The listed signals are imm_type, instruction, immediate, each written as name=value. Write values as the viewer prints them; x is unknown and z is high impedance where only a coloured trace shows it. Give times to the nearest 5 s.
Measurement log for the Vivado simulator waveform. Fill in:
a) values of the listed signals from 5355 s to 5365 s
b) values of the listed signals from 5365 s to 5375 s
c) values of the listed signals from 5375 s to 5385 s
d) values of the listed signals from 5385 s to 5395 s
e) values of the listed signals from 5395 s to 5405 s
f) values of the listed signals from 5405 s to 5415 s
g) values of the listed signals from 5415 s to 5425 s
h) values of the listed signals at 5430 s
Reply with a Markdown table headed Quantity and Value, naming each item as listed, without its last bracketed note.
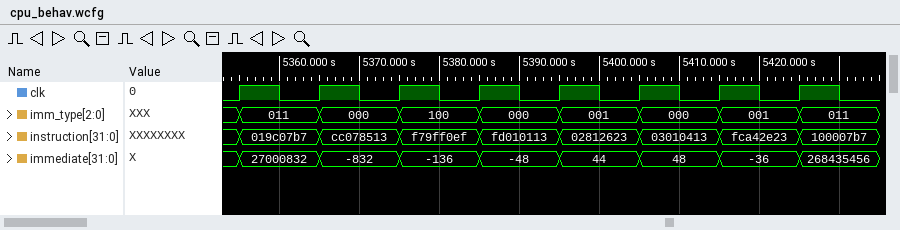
| Quantity | Value |
|---|---|
| values of the listed signals from 5355 s to 5365 s | imm_type=011, instruction=019c07b7, immediate=27000832 |
| values of the listed signals from 5365 s to 5375 s | imm_type=000, instruction=cc078513, immediate=-832 |
| values of the listed signals from 5375 s to 5385 s | imm_type=100, instruction=f79ff0ef, immediate=-136 |
| values of the listed signals from 5385 s to 5395 s | imm_type=000, instruction=fd010113, immediate=-48 |
| values of the listed signals from 5395 s to 5405 s | imm_type=001, instruction=02812623, immediate=44 |
| values of the listed signals from 5405 s to 5415 s | imm_type=000, instruction=03010413, immediate=48 |
| values of the listed signals from 5415 s to 5425 s | imm_type=001, instruction=fca42e23, immediate=-36 |
| values of the listed signals at 5430 s | imm_type=011, instruction=100007b7, immediate=268435456 |
